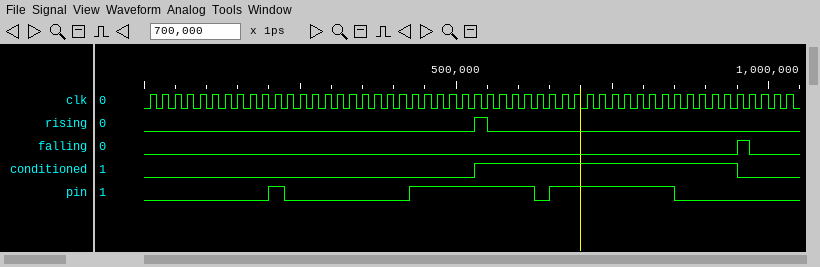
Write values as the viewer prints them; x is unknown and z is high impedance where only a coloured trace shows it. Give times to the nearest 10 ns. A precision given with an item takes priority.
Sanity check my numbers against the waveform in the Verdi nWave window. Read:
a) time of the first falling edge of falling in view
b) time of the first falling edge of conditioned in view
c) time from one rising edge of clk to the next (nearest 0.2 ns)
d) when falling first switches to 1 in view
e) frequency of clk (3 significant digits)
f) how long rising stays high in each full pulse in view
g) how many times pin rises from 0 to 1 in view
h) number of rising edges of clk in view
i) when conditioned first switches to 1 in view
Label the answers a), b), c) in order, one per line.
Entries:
a) 970 ns
b) 950 ns
c) 20 ns
d) 950 ns
e) 50.0 MHz
f) 20 ns
g) 3
h) 52
i) 530 ns
